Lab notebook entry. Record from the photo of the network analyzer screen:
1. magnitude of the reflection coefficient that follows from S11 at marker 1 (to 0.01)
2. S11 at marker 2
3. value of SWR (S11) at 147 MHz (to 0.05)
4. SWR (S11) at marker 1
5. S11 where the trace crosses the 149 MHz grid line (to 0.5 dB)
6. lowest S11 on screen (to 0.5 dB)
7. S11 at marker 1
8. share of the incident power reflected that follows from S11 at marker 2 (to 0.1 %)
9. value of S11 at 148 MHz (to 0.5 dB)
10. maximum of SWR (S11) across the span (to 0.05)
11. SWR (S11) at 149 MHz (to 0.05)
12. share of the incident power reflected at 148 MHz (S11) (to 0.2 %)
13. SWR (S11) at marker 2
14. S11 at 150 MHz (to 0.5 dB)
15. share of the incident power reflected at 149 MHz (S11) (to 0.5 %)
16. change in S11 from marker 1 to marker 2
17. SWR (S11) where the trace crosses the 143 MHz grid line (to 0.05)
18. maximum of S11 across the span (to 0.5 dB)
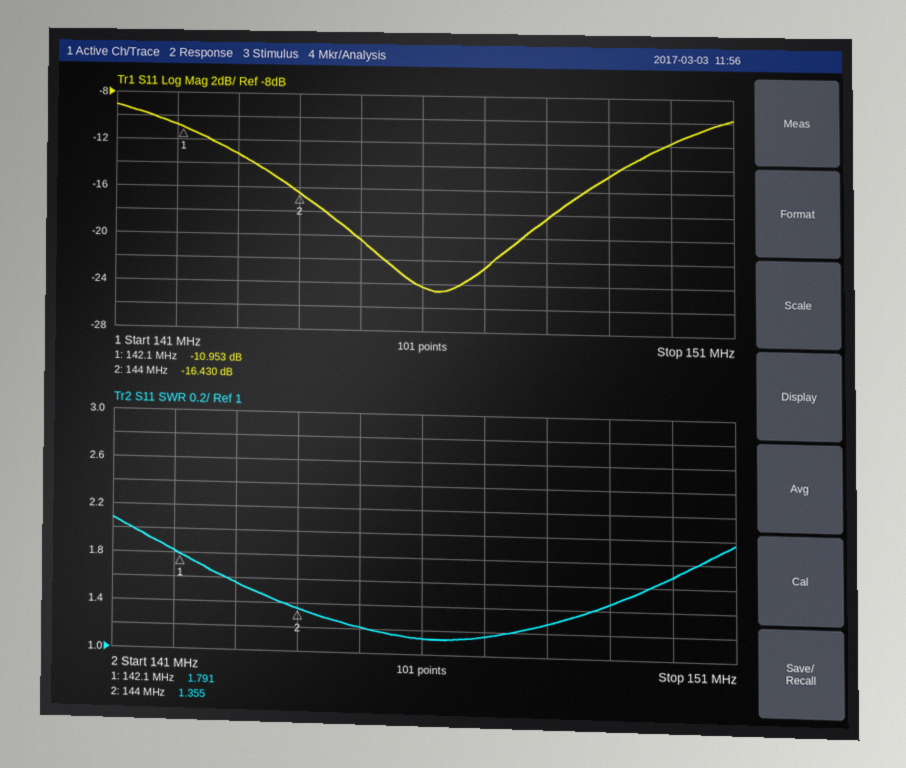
0.28
-16.430 dB
1.15
1.791
-14.5 dB
-24.5 dB
-10.953 dB
2.3 %
-18.5 dB
2.10
1.45
1.4 %
1.355
-12.0 dB
3.5 %
-5.477 dB
1.55
-9.0 dB
